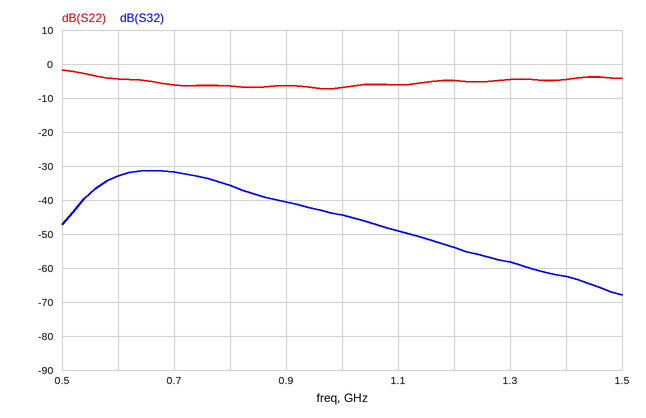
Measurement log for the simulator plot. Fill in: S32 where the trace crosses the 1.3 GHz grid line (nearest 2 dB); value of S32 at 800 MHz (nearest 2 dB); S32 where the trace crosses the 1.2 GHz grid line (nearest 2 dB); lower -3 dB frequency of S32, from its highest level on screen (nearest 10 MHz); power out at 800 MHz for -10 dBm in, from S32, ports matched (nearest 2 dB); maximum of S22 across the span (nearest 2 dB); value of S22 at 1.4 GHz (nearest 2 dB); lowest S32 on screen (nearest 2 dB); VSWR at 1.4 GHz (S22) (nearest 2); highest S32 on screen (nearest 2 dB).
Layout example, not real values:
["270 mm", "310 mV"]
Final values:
["-58 dB", "-36 dB", "-54 dB", "580 MHz", "-46 dBm", "-2 dB", "-4 dB", "-68 dB", "4", "-32 dB"]
